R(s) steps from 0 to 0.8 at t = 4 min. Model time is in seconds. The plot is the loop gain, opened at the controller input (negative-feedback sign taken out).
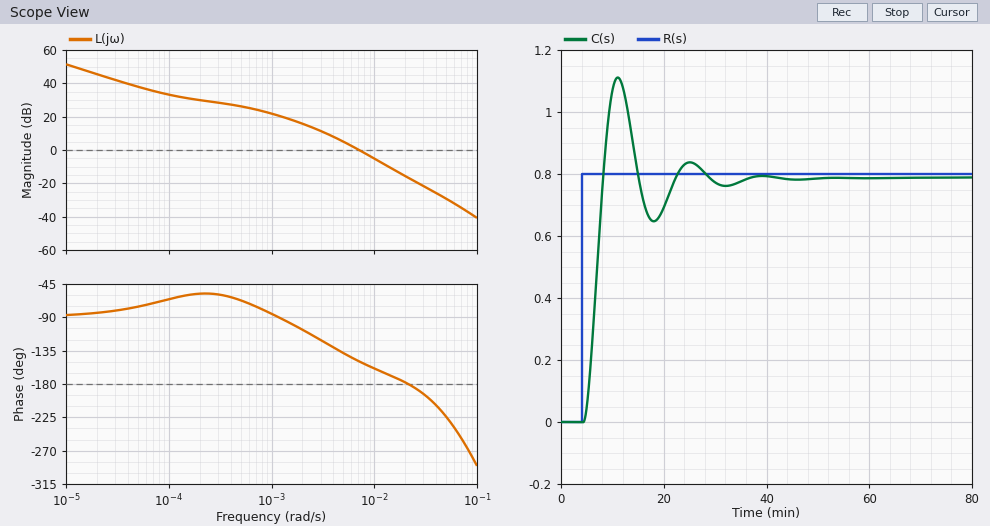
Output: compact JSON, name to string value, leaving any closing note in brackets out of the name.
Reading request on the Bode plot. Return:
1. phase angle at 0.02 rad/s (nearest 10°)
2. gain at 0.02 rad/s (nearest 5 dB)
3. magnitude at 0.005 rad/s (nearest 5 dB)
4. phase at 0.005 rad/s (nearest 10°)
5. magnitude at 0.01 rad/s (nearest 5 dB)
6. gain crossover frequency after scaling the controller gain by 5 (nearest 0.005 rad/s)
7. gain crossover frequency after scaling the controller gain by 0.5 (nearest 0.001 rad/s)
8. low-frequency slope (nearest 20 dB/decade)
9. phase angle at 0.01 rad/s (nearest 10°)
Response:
{"phase angle at 0.02 rad/s": "-180°", "gain at 0.02 rad/s": "-15 dB", "magnitude at 0.005 rad/s": "5 dB", "phase at 0.005 rad/s": "-140°", "magnitude at 0.01 rad/s": "-5 dB", "gain crossover frequency after scaling the controller gain by 5": "0.020 rad/s", "gain crossover frequency after scaling the controller gain by 0.5": "0.005 rad/s", "low-frequency slope": "-20 dB/decade", "phase angle at 0.01 rad/s": "-160°"}
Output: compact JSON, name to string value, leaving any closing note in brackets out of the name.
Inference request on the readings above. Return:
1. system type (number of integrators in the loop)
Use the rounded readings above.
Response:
{"system type": "1"}
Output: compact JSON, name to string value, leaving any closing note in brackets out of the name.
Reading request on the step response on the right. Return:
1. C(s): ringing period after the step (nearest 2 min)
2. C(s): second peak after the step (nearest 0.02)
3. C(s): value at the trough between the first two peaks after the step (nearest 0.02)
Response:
{"C(s): ringing period after the step": "14 min", "C(s): second peak after the step": "0.84", "C(s): value at the trough between the first two peaks after the step": "0.64"}
